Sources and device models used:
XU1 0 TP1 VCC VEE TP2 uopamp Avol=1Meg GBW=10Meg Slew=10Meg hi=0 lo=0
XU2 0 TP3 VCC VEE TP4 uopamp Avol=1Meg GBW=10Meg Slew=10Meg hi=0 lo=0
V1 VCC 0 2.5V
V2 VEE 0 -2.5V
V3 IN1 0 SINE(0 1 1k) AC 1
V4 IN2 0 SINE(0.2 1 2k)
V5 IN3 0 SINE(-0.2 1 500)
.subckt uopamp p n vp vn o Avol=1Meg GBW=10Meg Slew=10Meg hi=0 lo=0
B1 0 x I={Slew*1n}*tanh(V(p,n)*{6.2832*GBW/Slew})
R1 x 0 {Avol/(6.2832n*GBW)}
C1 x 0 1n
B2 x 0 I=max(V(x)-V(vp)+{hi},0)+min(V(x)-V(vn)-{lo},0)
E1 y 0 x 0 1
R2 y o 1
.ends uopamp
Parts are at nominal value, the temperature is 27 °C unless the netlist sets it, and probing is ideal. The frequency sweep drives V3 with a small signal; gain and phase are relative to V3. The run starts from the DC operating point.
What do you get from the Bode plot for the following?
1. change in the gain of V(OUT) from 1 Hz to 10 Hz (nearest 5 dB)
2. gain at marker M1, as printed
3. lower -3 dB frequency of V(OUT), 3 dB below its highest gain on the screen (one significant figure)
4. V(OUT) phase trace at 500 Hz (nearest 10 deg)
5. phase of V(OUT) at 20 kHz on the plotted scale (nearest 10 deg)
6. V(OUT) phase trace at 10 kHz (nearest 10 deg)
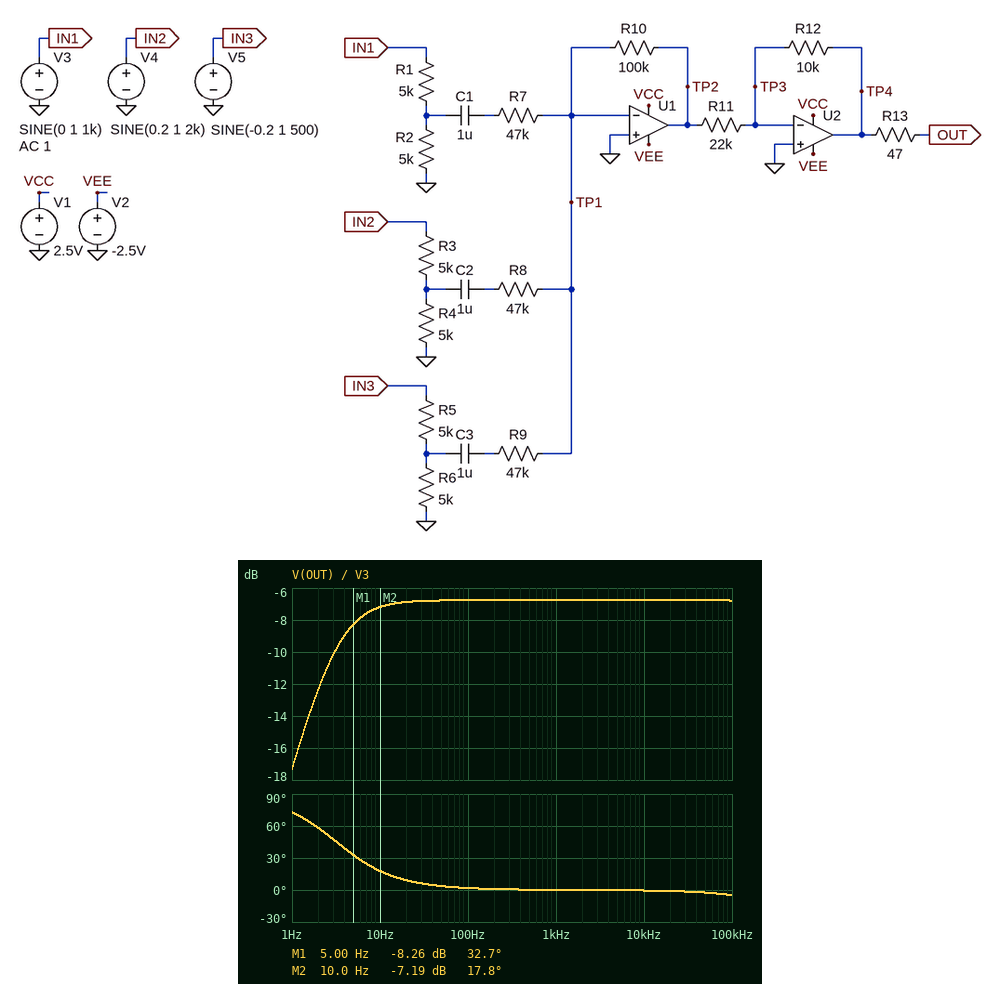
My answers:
10 dB
-8.26 dB
3 Hz
0 deg
0 deg
0 deg
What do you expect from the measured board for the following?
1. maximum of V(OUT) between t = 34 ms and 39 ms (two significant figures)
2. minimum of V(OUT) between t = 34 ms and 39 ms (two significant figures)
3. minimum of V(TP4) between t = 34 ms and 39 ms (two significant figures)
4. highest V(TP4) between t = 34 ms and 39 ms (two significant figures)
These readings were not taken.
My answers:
1.0 V
-1.0 V
-1.0 V
1.0 V
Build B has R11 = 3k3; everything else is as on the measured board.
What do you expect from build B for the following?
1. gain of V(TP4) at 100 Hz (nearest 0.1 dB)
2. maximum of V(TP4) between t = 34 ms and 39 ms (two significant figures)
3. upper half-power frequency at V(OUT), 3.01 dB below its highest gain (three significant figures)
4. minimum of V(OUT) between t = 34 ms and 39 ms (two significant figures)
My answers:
9.7 dB
2.5 V
1.14 MHz
-2.5 V
